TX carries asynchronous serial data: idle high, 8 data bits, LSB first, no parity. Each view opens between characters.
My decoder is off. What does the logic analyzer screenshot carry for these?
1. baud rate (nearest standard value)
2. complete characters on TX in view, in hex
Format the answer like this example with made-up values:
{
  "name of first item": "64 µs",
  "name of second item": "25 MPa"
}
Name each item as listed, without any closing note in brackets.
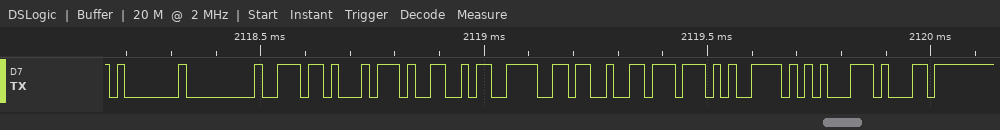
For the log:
{
  "baud rate": "57600 baud",
  "complete characters on TX in view, in hex": "01, 00, 6E, 74, A6, 9E, 93, 77, 79, C5, B1"
}
